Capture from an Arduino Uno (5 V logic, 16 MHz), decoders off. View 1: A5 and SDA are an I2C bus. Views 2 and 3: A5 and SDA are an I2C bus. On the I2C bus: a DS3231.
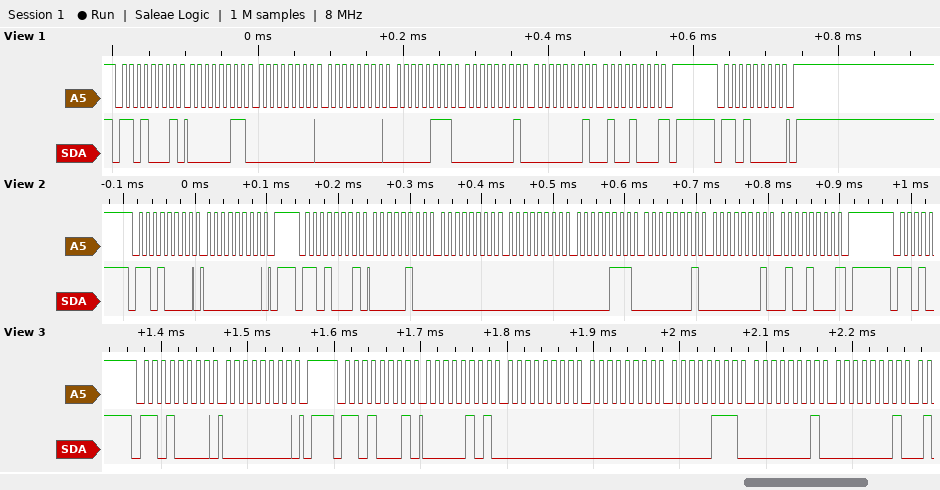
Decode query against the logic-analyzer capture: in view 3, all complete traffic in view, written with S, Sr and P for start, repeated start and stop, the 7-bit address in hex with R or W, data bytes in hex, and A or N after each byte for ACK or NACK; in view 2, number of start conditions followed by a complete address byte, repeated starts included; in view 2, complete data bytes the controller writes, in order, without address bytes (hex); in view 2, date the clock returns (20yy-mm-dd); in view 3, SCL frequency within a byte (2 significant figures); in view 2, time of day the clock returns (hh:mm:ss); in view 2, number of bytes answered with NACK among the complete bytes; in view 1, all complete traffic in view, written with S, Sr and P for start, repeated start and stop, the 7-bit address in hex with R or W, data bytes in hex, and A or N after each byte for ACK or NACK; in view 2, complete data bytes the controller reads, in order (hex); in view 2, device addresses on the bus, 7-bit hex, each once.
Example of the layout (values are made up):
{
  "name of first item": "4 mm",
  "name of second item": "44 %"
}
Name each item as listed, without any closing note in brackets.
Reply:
{
  "in view 3, all complete traffic in view, written with S, Sr and P for start, repeated start and stop, the 7-bit address in hex with R or W, data bytes in hex, and A or N after each byte for ACK or NACK": "S 68W A 00 A P S 68R A 05 A 00 A 00 A 07 A 01 A 01 A",
  "in view 2, number of start conditions followed by a complete address byte, repeated starts included": "2",
  "in view 2, complete data bytes the controller writes, in order, without address bytes": "00",
  "in view 2, date the clock returns": "2048-01-01",
  "in view 3, SCL frequency within a byte": "100 kHz",
  "in view 2, time of day the clock returns": "00:00:04",
  "in view 2, number of bytes answered with NACK among the complete bytes": "1",
  "in view 1, all complete traffic in view, written with S, Sr and P for start, repeated start and stop, the 7-bit address in hex with R or W, data bytes in hex, and A or N after each byte for ACK or NACK": "S 68R A 03 A 00 A 00 A 07 A 01 A 01 A 48 N P S 68W A P",
  "in view 2, complete data bytes the controller reads, in order": "04 00 00 07 01 01 48",
  "in view 2, device addresses on the bus, 7-bit hex, each once": "0x68"
}
